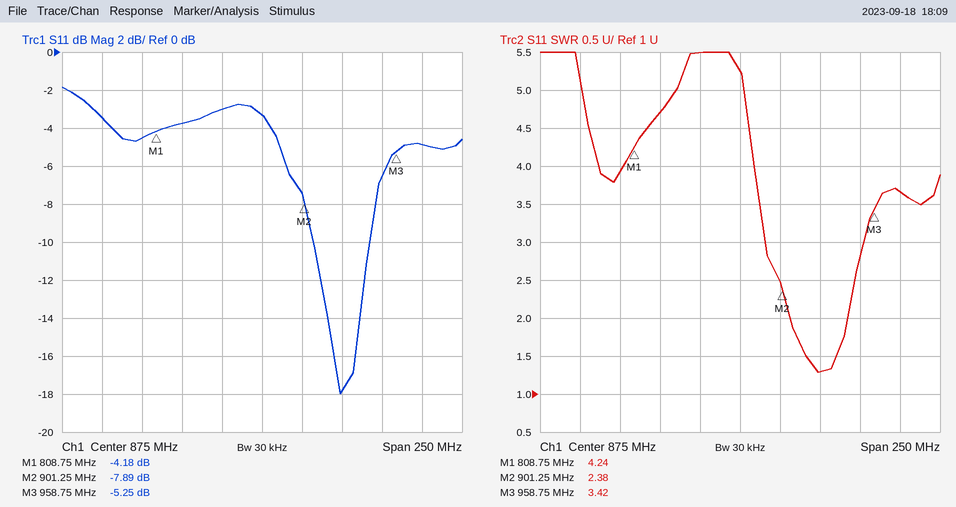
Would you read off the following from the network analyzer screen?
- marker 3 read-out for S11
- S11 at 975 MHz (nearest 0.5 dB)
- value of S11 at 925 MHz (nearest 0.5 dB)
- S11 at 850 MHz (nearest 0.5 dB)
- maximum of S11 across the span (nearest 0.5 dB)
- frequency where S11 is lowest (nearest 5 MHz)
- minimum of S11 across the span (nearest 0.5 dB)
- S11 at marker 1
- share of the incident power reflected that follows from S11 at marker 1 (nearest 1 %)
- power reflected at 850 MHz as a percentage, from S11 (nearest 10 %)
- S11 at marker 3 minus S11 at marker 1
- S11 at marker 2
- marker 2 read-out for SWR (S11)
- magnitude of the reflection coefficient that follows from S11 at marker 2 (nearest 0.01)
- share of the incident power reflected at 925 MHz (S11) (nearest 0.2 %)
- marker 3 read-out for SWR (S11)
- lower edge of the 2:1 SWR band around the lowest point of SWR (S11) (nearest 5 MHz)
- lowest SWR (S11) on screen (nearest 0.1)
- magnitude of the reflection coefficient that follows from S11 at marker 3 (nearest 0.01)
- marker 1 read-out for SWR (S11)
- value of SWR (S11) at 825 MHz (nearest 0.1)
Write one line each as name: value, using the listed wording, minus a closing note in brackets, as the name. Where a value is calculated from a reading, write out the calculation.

marker 3 read-out for S11: -5.25 dB
S11 at 975 MHz: -5.0 dB
value of S11 at 925 MHz: -18.0 dB
S11 at 850 MHz: -3.0 dB
maximum of S11 across the span: -2.0 dB
frequency where S11 is lowest: 925 MHz
minimum of S11 across the span: -18.0 dB
S11 at marker 1: -4.18 dB
share of the incident power reflected that follows from S11 at marker 1: 10^(-4.18/10) ≈ 38 %
power reflected at 850 MHz as a percentage, from S11: 10^(-3/10) ≈ 50 %
S11 at marker 3 minus S11 at marker 1: -5.25 − (-4.18) = -1.07 dB
S11 at marker 2: -7.89 dB
marker 2 read-out for SWR: 2.38
magnitude of the reflection coefficient that follows from S11 at marker 2: 10^(-7.89/20) ≈ 0.40
share of the incident power reflected at 925 MHz (S11): 10^(-18/10) ≈ 1.6 %
marker 3 read-out for SWR: 3.42
lower edge of the 2:1 SWR band around the lowest point of SWR (S11): 905 MHz
lowest SWR (S11) on screen: 1.3
magnitude of the reflection coefficient that follows from S11 at marker 3: 10^(-5.25/20) ≈ 0.55
marker 1 read-out for SWR: 4.24
value of SWR (S11) at 825 MHz: 4.7
